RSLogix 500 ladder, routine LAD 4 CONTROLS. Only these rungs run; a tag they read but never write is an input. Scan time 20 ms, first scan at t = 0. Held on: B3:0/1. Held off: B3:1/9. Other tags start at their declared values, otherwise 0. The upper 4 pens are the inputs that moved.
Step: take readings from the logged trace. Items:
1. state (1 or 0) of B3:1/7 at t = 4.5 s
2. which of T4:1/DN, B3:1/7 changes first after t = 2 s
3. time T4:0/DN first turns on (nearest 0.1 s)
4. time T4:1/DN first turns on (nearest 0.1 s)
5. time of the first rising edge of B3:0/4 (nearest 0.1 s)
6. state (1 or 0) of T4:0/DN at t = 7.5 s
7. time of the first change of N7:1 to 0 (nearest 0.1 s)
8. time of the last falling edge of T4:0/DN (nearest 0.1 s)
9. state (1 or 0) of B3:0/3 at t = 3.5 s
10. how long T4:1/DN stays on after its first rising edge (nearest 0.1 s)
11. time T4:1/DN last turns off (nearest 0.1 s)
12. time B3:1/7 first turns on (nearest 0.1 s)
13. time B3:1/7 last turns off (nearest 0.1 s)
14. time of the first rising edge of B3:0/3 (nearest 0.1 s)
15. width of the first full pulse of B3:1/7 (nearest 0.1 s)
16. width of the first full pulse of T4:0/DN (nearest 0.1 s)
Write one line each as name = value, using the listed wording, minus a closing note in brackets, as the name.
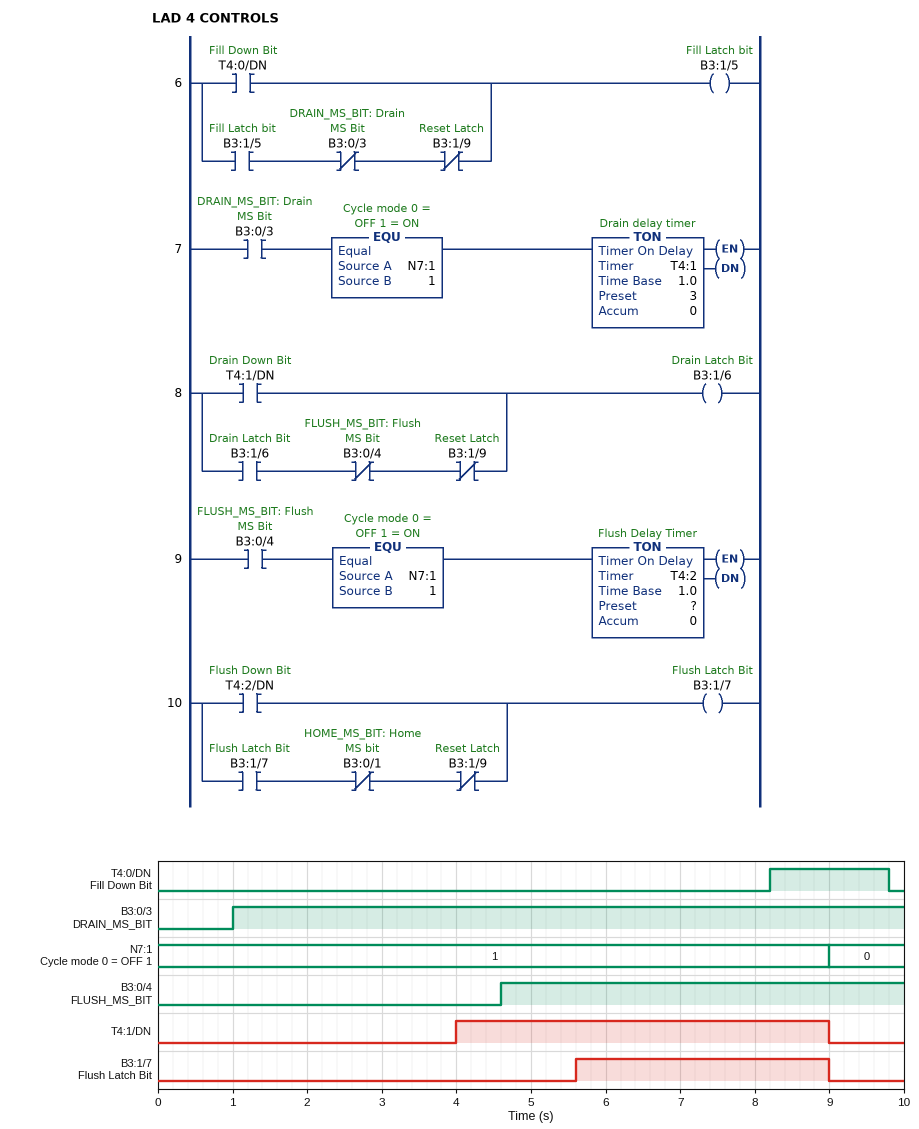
state (1 or 0) of B3:1/7 at t = 4.5 s = 0
which of T4:1/DN, B3:1/7 changes first after t = 2 s = T4:1/DN
time T4:0/DN first turns on = 8.2 s
time T4:1/DN first turns on = 4.0 s
time of the first rising edge of B3:0/4 = 4.6 s
state (1 or 0) of T4:0/DN at t = 7.5 s = 0
time of the first change of N7:1 to 0 = 9.0 s
time of the last falling edge of T4:0/DN = 9.8 s
state (1 or 0) of B3:0/3 at t = 3.5 s = 1
how long T4:1/DN stays on after its first rising edge = 5.0 s
time T4:1/DN last turns off = 9.0 s
time B3:1/7 first turns on = 5.6 s
time B3:1/7 last turns off = 9.0 s
time of the first rising edge of B3:0/3 = 1.0 s
width of the first full pulse of B3:1/7 = 3.4 s
width of the first full pulse of T4:0/DN = 1.6 s
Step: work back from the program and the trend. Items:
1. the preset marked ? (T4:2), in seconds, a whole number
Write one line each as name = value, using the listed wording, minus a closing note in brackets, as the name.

the preset marked ? (T4:2), in seconds, a whole number = 1 s
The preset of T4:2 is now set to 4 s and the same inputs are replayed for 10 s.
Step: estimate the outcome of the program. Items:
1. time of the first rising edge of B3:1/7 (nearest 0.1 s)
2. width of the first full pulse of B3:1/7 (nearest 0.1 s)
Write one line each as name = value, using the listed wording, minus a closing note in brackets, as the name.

time of the first rising edge of B3:1/7 = 8.6 s
width of the first full pulse of B3:1/7 = 0.4 s
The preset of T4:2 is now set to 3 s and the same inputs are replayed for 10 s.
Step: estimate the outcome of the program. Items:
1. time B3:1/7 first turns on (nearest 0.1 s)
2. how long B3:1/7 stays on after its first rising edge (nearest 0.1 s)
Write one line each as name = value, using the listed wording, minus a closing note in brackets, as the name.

time B3:1/7 first turns on = 7.6 s
how long B3:1/7 stays on after its first rising edge = 1.4 s
